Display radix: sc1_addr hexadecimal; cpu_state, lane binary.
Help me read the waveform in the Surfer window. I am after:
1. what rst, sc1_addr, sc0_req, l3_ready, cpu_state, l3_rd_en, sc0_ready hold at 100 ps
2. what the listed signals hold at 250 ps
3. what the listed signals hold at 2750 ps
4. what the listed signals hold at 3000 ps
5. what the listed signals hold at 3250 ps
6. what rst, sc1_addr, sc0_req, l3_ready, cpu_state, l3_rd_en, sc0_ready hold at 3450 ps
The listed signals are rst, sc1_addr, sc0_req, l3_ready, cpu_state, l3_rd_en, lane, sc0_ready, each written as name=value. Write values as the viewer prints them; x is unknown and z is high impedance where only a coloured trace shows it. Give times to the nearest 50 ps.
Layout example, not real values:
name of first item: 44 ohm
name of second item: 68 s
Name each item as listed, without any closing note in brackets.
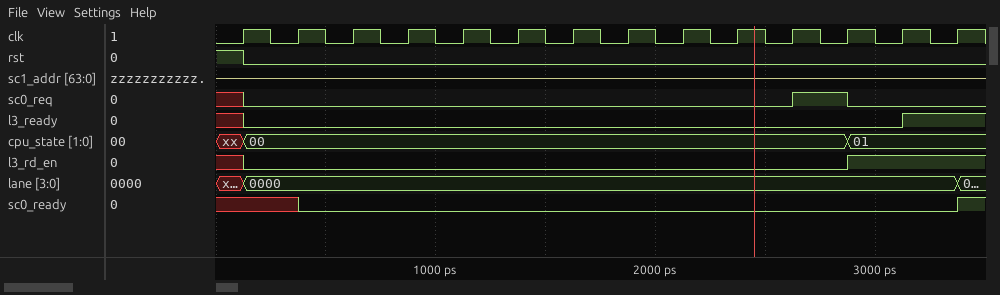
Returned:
what rst, sc1_addr, sc0_req, l3_ready, cpu_state, l3_rd_en, sc0_ready hold at 100 ps: rst=1, sc1_addr=z, sc0_req=x, l3_ready=x, cpu_state=xx, l3_rd_en=x, sc0_ready=x
what the listed signals hold at 250 ps: rst=0, sc1_addr=z, sc0_req=0, l3_ready=0, cpu_state=00, l3_rd_en=0, lane=0000, sc0_ready=x
what the listed signals hold at 2750 ps: rst=0, sc1_addr=z, sc0_req=1, l3_ready=0, cpu_state=00, l3_rd_en=0, lane=0000, sc0_ready=0
what the listed signals hold at 3000 ps: rst=0, sc1_addr=z, sc0_req=0, l3_ready=0, cpu_state=01, l3_rd_en=1, lane=0000, sc0_ready=0
what the listed signals hold at 3250 ps: rst=0, sc1_addr=z, sc0_req=0, l3_ready=1, cpu_state=01, l3_rd_en=1, lane=0000, sc0_ready=0
what rst, sc1_addr, sc0_req, l3_ready, cpu_state, l3_rd_en, sc0_ready hold at 3450 ps: rst=0, sc1_addr=z, sc0_req=0, l3_ready=1, cpu_state=01, l3_rd_en=1, sc0_ready=1
